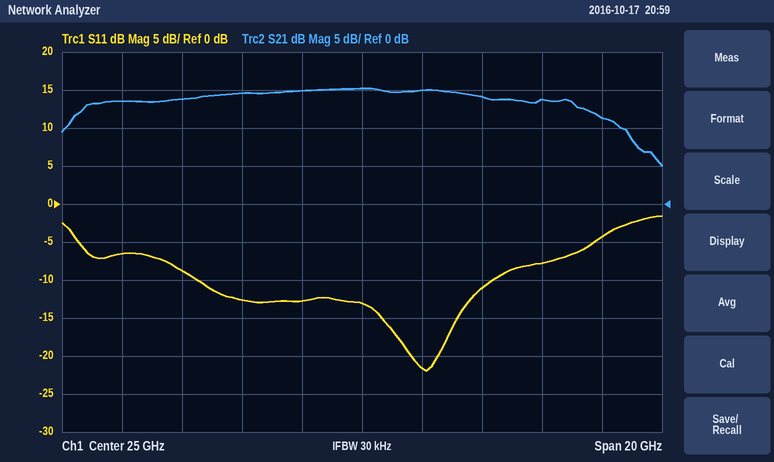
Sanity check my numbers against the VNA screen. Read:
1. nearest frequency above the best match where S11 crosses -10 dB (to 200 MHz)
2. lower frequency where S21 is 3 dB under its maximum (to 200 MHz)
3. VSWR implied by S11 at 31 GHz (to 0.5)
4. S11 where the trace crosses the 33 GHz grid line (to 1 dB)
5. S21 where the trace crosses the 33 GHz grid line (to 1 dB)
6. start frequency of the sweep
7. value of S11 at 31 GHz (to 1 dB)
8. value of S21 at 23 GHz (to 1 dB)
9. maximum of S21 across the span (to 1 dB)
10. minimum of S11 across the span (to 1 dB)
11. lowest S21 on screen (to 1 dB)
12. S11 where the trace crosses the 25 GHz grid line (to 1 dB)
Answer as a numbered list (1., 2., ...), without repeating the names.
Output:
1. 29.4 GHz
2. 15.6 GHz
3. 2.5
4. -4 dB
5. 11 dB
6. 15 GHz
7. -8 dB
8. 15 dB
9. 15 dB
10. -22 dB
11. 5 dB
12. -13 dB
